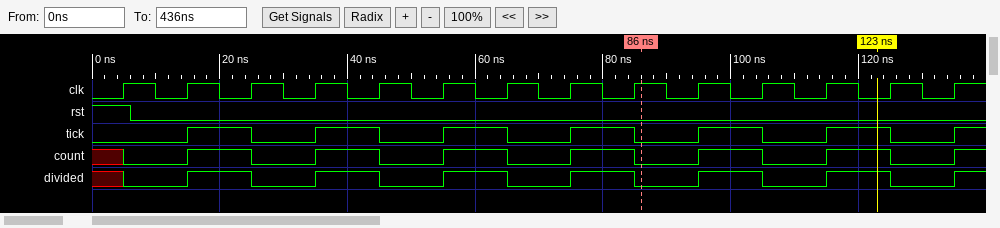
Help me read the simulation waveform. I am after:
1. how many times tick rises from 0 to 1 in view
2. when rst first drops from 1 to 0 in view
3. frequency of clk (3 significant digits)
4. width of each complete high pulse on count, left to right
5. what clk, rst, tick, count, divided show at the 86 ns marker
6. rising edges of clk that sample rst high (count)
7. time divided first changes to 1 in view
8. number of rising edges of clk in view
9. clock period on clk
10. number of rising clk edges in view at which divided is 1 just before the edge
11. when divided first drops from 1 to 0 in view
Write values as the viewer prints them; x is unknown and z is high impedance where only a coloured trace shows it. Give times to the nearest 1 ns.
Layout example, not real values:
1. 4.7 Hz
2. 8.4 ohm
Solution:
1. 7
2. 6 ns
3. 100 MHz
4. 10 ns, 10 ns, 10 ns, 10 ns, 10 ns, 10 ns
5. clk=1, rst=0, tick=0, count=0, divided=0
6. 1
7. 15 ns
8. 14
9. 10 ns
10. 6
11. 25 ns
